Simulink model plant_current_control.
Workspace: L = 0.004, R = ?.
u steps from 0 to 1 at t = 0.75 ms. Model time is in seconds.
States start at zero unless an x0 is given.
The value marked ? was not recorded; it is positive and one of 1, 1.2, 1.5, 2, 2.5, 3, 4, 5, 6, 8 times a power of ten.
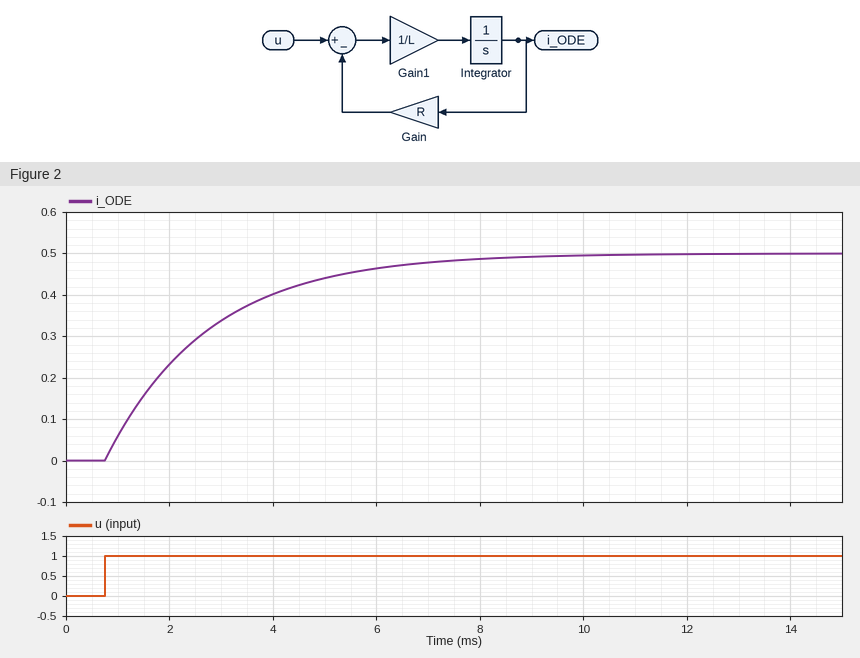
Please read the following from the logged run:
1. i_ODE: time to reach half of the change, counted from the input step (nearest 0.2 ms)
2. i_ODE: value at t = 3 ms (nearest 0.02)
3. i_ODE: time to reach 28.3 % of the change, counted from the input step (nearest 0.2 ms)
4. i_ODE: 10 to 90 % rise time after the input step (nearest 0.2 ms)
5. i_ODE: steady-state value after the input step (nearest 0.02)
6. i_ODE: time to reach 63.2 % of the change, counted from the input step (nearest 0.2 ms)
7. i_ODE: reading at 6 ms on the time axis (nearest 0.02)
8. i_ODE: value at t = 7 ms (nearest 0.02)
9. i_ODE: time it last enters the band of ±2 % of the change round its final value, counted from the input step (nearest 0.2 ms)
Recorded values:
1.4 ms
0.34
0.6 ms
4.4 ms
0.50
2.0 ms
0.46
0.48
7.8 ms
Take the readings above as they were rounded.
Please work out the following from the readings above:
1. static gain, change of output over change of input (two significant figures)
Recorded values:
0.50
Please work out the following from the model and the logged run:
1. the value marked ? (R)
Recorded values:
2
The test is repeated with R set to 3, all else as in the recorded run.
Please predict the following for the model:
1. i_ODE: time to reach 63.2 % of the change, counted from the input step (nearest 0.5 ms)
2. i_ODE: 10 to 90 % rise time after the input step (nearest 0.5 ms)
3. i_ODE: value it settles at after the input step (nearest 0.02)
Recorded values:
1.5 ms
3.0 ms
0.34
